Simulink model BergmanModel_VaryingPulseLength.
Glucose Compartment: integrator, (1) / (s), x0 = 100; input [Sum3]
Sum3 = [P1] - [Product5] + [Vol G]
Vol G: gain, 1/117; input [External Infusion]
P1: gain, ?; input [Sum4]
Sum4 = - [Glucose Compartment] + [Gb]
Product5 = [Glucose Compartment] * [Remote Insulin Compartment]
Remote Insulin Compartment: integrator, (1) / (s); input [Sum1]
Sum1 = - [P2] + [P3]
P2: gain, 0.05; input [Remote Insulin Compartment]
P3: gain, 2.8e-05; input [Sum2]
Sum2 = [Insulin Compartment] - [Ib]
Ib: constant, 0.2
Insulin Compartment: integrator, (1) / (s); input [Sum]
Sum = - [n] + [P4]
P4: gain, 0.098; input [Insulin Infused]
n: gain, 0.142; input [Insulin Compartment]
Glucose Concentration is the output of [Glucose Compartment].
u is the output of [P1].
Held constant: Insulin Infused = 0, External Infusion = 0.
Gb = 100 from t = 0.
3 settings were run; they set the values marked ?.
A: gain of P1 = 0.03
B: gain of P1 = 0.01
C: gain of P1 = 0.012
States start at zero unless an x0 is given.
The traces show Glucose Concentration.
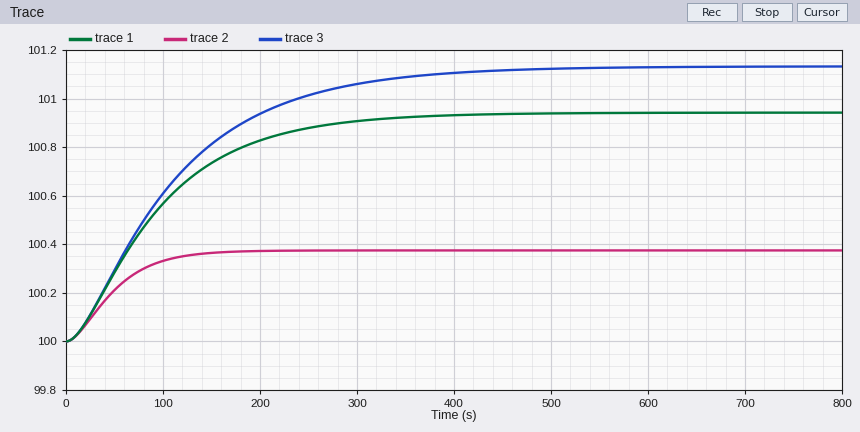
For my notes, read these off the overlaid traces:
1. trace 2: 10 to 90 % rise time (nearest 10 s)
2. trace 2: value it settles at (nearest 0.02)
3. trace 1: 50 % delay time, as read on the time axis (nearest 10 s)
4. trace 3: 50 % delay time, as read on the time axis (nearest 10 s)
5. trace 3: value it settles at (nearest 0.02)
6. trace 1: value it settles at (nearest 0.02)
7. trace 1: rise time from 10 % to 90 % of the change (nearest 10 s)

90 s
100.38
80 s
90 s
101.14
100.94
190 s
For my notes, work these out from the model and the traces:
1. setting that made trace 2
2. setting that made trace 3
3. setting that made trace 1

A
B
C
